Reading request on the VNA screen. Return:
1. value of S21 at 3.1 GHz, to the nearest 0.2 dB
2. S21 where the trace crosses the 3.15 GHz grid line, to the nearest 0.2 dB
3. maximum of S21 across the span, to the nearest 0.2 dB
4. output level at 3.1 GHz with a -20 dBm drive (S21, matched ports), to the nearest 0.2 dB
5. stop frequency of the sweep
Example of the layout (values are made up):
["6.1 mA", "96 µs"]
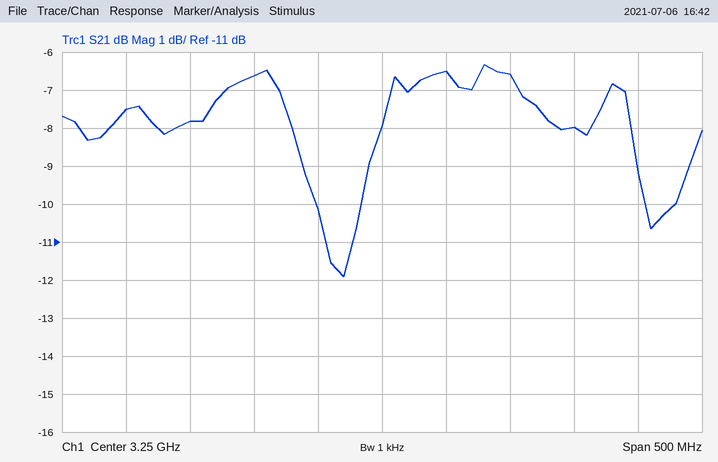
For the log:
["-7.8 dB", "-6.6 dB", "-6.4 dB", "-27.8 dBm", "3.5 GHz"]
